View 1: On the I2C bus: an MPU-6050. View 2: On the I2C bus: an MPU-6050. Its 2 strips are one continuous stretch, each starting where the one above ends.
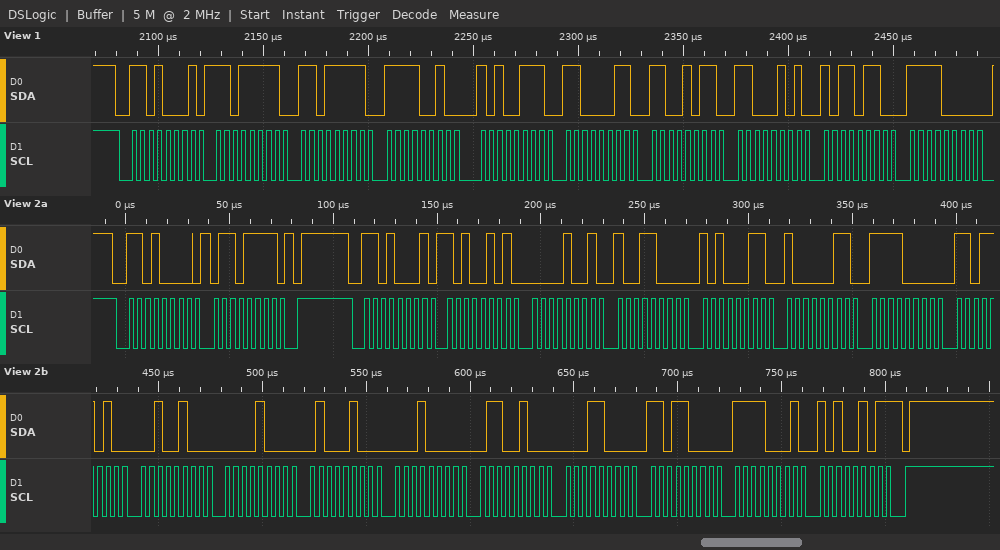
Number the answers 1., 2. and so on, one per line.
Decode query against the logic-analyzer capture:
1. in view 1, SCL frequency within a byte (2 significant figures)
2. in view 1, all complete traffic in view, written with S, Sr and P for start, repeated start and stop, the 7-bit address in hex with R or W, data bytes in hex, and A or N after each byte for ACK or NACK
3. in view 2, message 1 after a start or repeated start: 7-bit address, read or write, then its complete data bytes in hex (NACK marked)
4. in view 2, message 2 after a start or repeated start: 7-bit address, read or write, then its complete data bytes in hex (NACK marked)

1. 250 kHz
2. S 68R A DF A DF A F2 A A7 A C3 A CB A C5 A B6 A F0 A
3. 0x68 write: 6F
4. 0x68 read: A5 09 98 A3 83 F0 DA 24 08 44 10 64 18 D8 F1 A5 NACK
